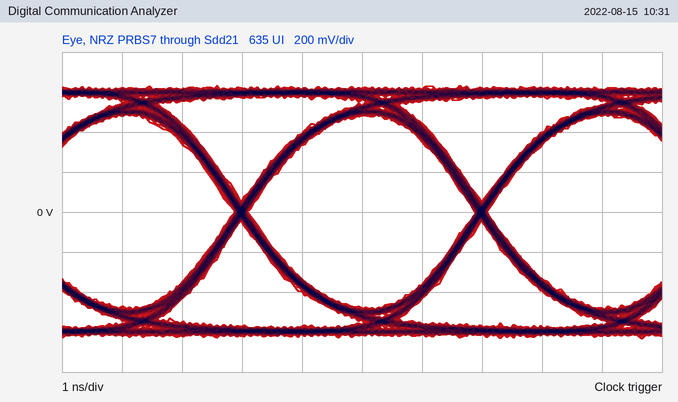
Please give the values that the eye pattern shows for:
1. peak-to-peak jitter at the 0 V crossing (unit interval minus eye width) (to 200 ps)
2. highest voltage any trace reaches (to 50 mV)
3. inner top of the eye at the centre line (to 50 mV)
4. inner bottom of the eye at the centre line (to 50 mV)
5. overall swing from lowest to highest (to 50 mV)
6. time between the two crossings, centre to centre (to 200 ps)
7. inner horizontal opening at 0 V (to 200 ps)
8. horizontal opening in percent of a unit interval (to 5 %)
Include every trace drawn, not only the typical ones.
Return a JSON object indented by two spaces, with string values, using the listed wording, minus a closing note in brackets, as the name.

{
  "peak-to-peak jitter at the 0 V crossing (unit interval minus eye width)": "200 ps",
  "highest voltage any trace reaches": "650 mV",
  "inner top of the eye at the centre line": "500 mV",
  "inner bottom of the eye at the centre line": "-500 mV",
  "overall swing from lowest to highest": "1.25 V",
  "time between the two crossings, centre to centre": "4.0 ns",
  "inner horizontal opening at 0 V": "3.8 ns",
  "horizontal opening in percent of a unit interval": "95 %"
}
